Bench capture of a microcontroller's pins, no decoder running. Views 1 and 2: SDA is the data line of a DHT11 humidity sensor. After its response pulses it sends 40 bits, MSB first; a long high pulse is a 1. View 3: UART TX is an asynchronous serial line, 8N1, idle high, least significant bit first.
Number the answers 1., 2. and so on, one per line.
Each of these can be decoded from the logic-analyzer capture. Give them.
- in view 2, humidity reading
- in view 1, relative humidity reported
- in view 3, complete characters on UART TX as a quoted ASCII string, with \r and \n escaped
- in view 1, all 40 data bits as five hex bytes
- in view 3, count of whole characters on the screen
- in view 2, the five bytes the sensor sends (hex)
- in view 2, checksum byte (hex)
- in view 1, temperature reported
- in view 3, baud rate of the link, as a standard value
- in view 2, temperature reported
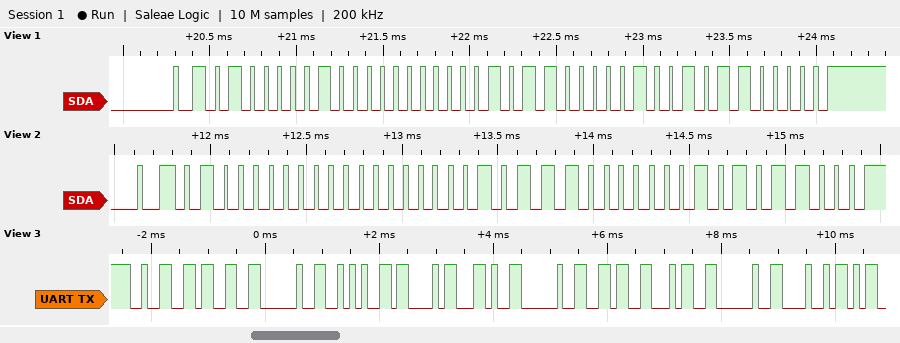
1. 64 %
2. 65 %
3. "23 *C, 64 H"
4. 41 00 16 09 60
5. 11
6. 40 00 17 01 58
7. 0x58
8. 22.9 °C
9. 9600 baud
10. 23.1 °C
